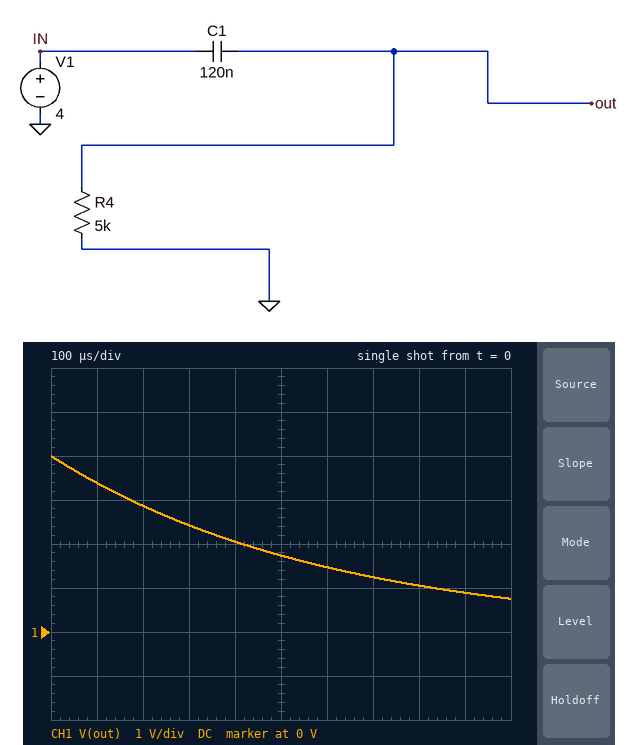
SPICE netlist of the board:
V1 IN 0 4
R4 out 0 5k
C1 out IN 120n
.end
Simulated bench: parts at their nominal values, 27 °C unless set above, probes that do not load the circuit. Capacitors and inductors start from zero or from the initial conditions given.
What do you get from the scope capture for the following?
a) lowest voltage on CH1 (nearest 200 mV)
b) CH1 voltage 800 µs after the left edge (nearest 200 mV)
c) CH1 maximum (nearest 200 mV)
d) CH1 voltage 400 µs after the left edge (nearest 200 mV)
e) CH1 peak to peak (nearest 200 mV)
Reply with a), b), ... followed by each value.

a) 800 mV
b) 1.0 V
c) 4.0 V
d) 2.0 V
e) 3.2 V
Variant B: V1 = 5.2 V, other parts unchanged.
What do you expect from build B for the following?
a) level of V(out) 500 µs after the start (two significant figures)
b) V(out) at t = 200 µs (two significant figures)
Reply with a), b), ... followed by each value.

a) 2.3 V
b) 3.7 V
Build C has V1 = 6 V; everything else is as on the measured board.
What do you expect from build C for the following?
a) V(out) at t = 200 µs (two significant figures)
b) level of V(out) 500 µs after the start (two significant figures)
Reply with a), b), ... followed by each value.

a) 4.3 V
b) 2.6 V
